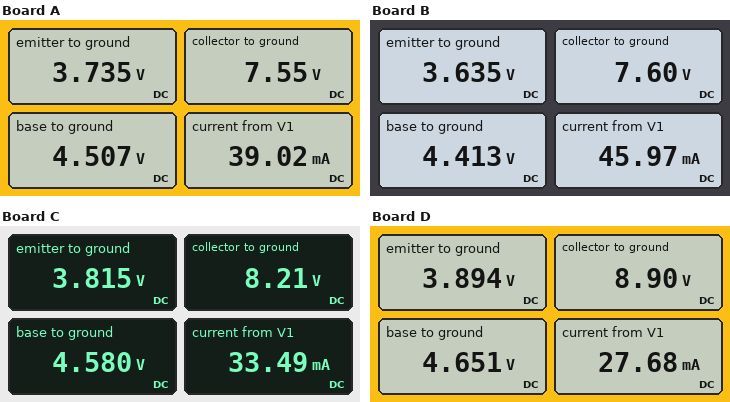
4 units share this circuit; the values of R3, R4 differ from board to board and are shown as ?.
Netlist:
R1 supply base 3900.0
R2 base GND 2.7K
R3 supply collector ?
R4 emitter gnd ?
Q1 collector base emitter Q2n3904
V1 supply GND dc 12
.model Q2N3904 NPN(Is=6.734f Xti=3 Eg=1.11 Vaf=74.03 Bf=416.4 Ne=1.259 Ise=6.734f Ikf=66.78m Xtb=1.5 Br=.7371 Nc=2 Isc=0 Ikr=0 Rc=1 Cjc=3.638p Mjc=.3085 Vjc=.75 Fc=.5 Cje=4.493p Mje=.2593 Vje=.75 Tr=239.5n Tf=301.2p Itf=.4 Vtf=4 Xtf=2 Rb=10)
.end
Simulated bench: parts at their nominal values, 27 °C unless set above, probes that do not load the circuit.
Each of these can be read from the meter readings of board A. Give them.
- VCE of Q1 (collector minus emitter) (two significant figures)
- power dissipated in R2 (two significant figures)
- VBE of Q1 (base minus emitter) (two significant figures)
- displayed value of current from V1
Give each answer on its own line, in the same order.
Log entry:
3.8 V
7.5 mW
770 mV
39.02 mA
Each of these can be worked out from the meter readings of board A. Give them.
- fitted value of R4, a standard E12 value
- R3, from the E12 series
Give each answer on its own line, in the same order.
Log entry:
100 Ω
120 Ω
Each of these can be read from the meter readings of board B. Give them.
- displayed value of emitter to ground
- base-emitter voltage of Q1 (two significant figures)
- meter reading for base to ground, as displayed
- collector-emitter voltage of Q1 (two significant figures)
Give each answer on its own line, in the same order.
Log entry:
3.635 V
780 mV
4.413 V
4.0 V
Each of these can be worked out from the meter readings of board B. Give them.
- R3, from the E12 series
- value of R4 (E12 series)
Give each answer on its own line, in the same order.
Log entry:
100 Ω
82 Ω
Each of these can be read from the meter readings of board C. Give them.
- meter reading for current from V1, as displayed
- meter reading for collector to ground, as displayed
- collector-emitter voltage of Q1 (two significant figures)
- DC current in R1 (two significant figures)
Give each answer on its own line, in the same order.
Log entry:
33.49 mA
8.21 V
4.4 V
1.9 mA
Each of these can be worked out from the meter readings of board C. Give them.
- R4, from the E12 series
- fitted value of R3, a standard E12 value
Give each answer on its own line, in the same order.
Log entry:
120 Ω
120 Ω
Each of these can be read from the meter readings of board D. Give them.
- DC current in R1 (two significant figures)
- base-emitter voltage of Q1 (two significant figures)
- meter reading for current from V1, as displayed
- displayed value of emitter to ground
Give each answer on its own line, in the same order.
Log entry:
1.9 mA
760 mV
27.68 mA
3.894 V
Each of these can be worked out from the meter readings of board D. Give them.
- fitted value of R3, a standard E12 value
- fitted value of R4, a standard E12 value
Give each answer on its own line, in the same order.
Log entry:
120 Ω
150 Ω
